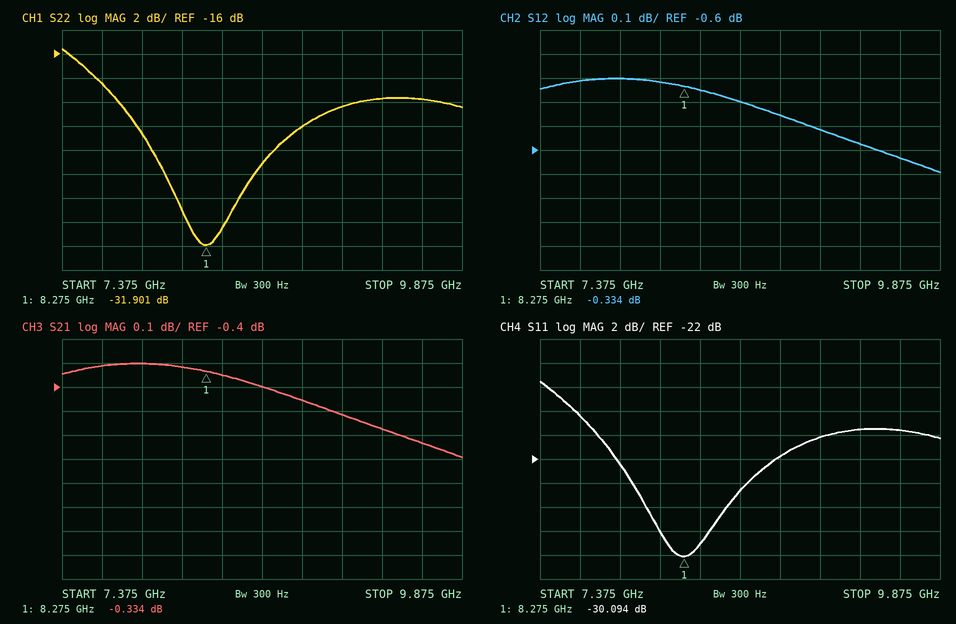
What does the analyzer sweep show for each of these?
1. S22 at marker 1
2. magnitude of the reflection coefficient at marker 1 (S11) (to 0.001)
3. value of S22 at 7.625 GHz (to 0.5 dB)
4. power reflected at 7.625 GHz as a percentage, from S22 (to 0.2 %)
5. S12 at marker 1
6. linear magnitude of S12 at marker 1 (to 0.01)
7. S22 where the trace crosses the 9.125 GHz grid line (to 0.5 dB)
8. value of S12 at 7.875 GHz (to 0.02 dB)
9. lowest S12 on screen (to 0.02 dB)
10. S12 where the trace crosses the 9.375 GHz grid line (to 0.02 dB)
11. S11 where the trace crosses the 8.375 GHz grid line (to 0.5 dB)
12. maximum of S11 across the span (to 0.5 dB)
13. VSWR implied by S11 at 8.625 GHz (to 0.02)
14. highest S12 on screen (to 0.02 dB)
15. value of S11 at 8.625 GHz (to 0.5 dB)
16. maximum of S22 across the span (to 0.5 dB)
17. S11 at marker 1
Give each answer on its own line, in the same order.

-31.901 dB
0.031
-18.5 dB
1.4 %
-0.334 dB
0.96
-20.5 dB
-0.30 dB
-0.70 dB
-0.58 dB
-29.0 dB
-15.5 dB
1.12
-0.30 dB
-24.5 dB
-15.5 dB
-30.094 dB
